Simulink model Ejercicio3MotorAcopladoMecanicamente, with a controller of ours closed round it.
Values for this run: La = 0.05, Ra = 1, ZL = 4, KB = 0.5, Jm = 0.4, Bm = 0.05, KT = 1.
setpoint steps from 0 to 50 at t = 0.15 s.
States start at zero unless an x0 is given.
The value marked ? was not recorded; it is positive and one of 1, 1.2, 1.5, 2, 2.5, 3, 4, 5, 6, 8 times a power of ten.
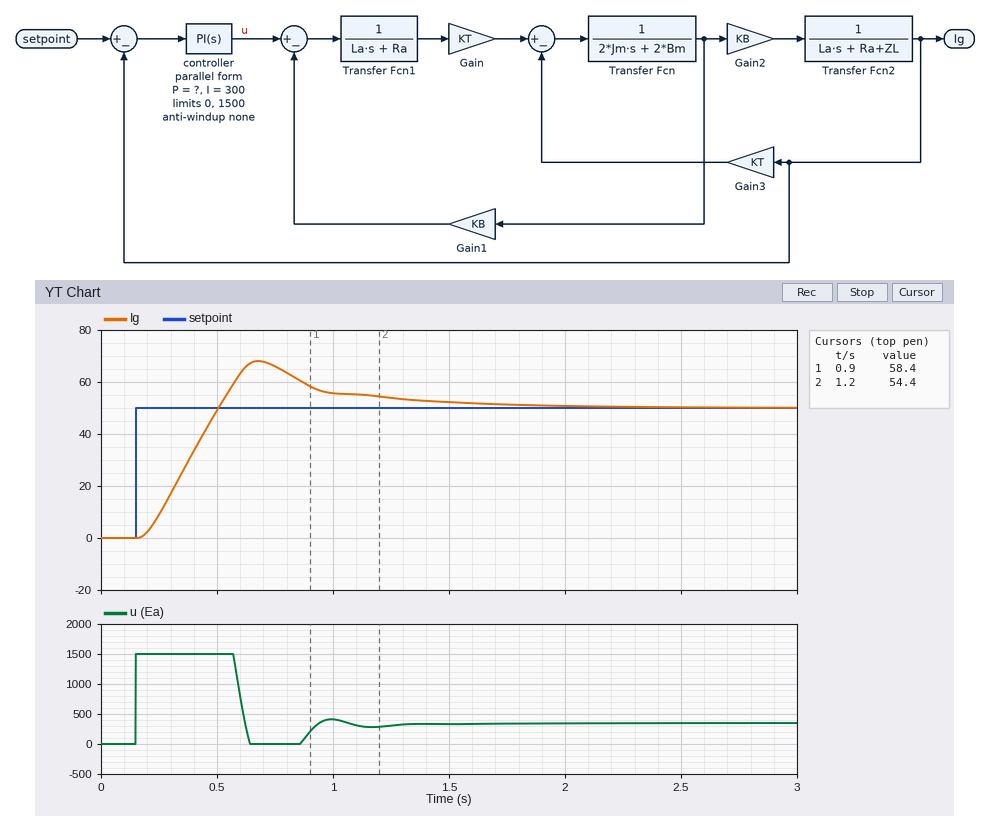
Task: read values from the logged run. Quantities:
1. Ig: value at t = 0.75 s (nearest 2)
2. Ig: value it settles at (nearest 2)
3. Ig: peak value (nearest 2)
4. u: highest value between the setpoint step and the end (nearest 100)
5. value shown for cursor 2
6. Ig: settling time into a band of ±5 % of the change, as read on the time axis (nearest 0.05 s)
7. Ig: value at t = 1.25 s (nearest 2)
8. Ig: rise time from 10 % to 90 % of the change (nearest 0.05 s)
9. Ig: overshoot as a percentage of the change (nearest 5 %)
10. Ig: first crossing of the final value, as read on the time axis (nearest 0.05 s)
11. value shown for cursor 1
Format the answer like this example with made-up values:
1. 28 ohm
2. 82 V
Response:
1. 66
2. 50
3. 68
4. 1500
5. 54.4
6. 1.45 s
7. 54
8. 0.25 s
9. 35 %
10. 0.50 s
11. 58.4
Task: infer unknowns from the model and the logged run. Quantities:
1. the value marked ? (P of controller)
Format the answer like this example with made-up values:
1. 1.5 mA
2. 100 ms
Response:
1. 150
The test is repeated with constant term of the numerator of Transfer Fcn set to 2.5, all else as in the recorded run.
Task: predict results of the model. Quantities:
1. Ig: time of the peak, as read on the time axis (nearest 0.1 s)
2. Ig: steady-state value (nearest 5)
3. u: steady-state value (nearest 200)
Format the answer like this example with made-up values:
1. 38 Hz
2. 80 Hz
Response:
1. 0.4 s
2. 50
3. 400
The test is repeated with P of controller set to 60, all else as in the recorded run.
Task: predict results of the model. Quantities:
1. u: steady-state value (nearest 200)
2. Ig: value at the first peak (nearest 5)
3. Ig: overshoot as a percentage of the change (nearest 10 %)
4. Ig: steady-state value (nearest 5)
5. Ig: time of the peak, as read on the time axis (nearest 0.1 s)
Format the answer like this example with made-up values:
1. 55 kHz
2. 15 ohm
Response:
1. 400
2. 80
3. 60 %
4. 50
5. 0.8 s
